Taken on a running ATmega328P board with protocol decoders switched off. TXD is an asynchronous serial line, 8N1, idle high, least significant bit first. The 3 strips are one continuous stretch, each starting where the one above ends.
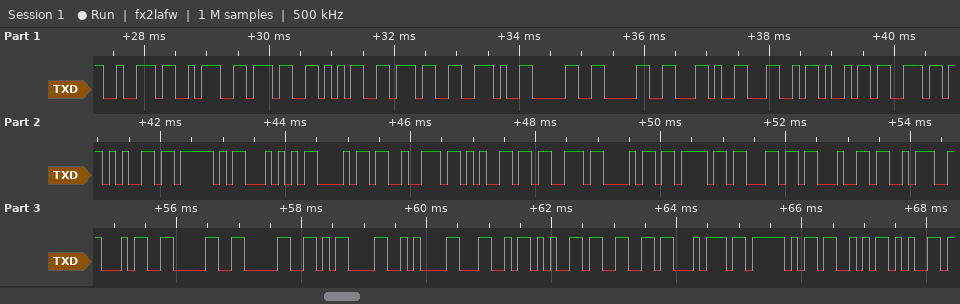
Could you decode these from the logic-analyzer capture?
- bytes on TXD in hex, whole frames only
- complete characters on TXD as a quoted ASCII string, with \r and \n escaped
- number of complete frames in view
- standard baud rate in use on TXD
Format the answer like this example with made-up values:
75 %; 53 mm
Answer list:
72 3A 37 35 37 2E 30 30 2C 4C 69 6E 65 5F 54 68 72 65 73 68 6F 6C 64 3A 34 30 30 0D 0A 4C 65 66 74 5F 53 65; "r:757.00,Line_Threshold:400\r\nLeft_Se"; 36; 9600 baud
